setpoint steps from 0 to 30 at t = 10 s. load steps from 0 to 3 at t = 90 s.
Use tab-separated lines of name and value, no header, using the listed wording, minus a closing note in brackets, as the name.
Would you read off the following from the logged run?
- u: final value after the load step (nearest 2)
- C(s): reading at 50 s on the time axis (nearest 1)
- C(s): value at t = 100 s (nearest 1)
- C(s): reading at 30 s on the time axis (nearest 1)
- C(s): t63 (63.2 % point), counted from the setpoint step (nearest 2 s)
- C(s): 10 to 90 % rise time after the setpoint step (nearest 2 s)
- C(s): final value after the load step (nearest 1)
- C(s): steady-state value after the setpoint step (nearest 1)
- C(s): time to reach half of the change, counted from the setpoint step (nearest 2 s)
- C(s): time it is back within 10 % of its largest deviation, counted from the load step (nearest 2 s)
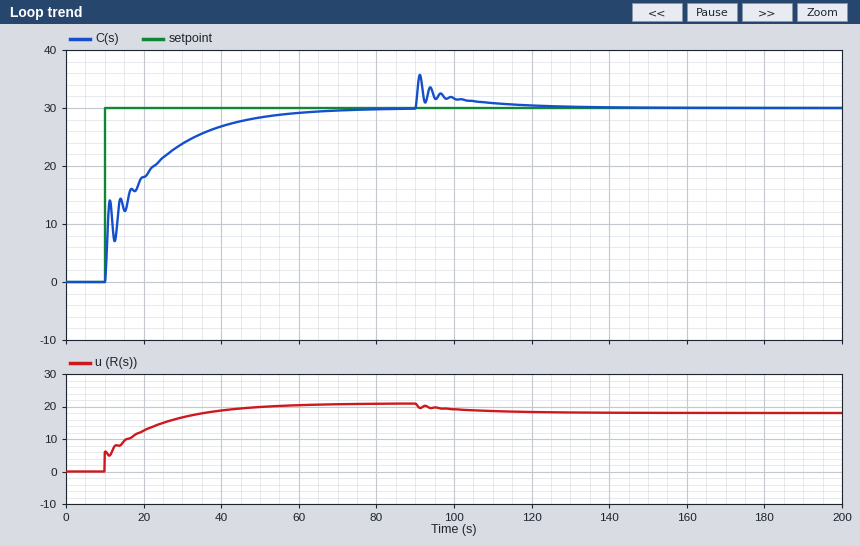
u: final value after the load step	18
C(s): reading at 50 s on the time axis	28
C(s): value at t = 100 s	32
C(s): reading at 30 s on the time axis	24
C(s): t63 (63.2 % point), counted from the setpoint step	12 s
C(s): 10 to 90 % rise time after the setpoint step	30 s
C(s): final value after the load step	30
C(s): steady-state value after the setpoint step	30
C(s): time to reach half of the change, counted from the setpoint step	6 s
C(s): time it is back within 10 % of its largest deviation, counted from the load step	26 s
